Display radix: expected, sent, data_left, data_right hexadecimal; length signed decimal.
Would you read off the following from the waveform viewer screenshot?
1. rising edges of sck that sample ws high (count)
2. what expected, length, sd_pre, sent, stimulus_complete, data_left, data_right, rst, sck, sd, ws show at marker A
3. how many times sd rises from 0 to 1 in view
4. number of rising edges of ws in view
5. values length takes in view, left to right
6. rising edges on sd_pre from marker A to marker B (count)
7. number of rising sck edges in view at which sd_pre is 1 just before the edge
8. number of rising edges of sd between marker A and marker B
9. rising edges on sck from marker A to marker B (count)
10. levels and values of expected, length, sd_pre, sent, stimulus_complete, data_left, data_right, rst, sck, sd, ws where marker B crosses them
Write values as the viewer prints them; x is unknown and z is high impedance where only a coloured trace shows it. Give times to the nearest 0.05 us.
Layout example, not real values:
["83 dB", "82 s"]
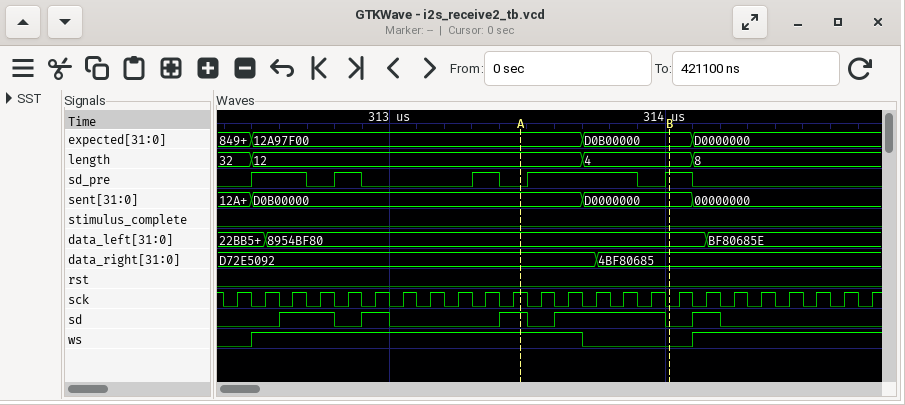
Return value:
["19", "expected=12A97F00, length=12, sd_pre=0, sent=D0B00000, stimulus_complete=0, data_left=8954BF80, data_right=D72E5092, rst=0, sck=1, sd=1, ws=1", "5", "2", "32, 12, 4, 8", "2", "9", "1", "5", "expected=D0B00000, length=4, sd_pre=1, sent=D0000000, stimulus_complete=0, data_left=8954BF80, data_right=4BF80685, rst=0, sck=0, sd=0, ws=0"]
